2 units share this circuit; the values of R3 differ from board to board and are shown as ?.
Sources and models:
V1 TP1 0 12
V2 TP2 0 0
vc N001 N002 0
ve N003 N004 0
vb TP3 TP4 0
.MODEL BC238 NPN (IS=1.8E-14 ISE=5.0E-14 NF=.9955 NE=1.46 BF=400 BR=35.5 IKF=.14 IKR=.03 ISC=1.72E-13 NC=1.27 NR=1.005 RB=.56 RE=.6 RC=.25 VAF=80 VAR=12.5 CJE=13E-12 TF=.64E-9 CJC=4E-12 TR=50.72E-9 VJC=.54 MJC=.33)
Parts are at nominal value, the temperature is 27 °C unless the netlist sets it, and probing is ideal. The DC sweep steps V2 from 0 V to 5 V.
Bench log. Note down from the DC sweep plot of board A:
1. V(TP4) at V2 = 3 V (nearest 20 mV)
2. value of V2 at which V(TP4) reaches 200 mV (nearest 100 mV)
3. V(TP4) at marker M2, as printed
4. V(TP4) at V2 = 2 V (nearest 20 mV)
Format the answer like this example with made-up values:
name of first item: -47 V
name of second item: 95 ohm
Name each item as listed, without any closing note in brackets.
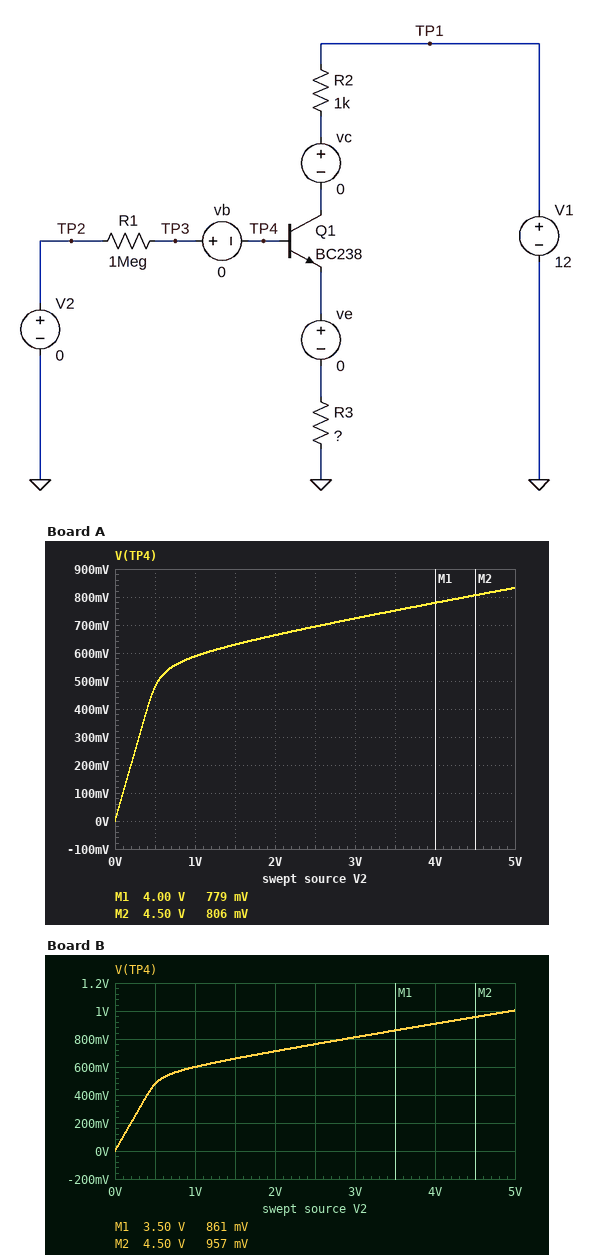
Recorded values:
V(TP4) at V2 = 3 V: 720 mV
value of V2 at which V(TP4) reaches 200 mV: 200 mV
V(TP4) at marker M2, as printed: 806 mV
V(TP4) at V2 = 2 V: 660 mV
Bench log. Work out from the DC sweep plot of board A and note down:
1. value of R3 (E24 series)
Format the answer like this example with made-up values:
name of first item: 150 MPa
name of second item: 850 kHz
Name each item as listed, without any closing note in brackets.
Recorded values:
value of R3: 150 Ω
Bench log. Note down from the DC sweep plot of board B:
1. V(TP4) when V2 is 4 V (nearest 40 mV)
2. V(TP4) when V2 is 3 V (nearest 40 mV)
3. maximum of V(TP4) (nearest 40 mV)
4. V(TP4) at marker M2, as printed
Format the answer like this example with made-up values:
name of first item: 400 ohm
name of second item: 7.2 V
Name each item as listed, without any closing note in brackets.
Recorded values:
V(TP4) when V2 is 4 V: 920 mV
V(TP4) when V2 is 3 V: 800 mV
maximum of V(TP4): 1.00 V
V(TP4) at marker M2, as printed: 957 mV
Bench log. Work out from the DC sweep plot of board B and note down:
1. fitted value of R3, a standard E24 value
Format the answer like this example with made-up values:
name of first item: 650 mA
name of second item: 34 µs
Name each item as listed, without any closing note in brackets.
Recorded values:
fitted value of R3, a standard E24 value: 300 Ω
